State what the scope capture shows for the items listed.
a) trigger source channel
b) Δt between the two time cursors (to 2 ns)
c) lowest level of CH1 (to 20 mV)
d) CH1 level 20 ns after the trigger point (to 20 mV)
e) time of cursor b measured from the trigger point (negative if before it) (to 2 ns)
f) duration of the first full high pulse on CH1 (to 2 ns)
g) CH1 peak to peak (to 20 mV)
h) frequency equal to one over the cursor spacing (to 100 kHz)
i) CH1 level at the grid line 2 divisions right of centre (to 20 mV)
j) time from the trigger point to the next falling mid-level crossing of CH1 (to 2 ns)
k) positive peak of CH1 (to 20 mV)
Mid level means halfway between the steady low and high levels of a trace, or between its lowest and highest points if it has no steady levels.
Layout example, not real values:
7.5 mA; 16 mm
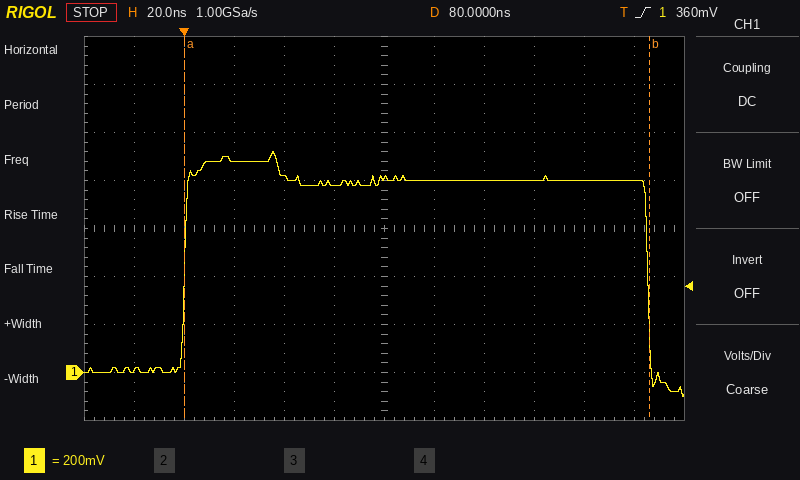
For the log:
CH1; 186 ns; -100 mV; 880 mV; +186 ns; 186 ns; 1.02 V; 5.4 MHz; 800 mV; 186 ns; 920 mV
